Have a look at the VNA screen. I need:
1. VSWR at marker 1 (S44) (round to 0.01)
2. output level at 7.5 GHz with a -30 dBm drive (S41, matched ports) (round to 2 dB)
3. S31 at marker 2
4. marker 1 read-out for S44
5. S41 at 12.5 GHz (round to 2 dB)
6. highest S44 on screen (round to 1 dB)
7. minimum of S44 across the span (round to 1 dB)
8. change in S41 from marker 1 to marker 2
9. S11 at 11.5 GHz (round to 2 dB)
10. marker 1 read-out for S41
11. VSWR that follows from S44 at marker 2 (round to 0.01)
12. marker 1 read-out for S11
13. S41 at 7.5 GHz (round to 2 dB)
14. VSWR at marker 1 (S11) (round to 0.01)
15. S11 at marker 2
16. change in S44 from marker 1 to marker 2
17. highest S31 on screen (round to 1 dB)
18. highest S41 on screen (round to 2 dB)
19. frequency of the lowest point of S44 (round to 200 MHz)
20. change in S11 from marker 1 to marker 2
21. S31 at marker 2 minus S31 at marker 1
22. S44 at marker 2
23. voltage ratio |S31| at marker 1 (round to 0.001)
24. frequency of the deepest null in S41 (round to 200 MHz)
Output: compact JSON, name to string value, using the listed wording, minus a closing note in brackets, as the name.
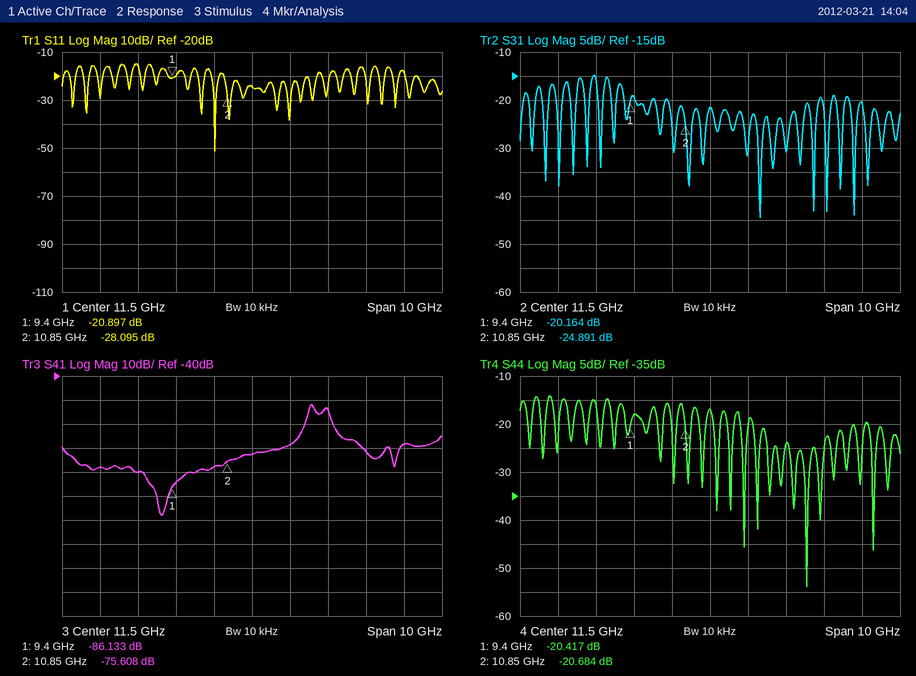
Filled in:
{"VSWR at marker 1 (S44)": "1.21", "output level at 7.5 GHz with a -30 dBm drive (S41, matched ports)": "-108 dBm", "S31 at marker 2": "-24.891 dB", "marker 1 read-out for S44": "-20.417 dB", "S41 at 12.5 GHz": "-68 dB", "highest S44 on screen": "-14 dB", "minimum of S44 across the span": "-54 dB", "change in S41 from marker 1 to marker 2": "10.525 dB", "S11 at 11.5 GHz": "-24 dB", "marker 1 read-out for S41": "-86.133 dB", "VSWR that follows from S44 at marker 2": "1.20", "marker 1 read-out for S11": "-20.897 dB", "S41 at 7.5 GHz": "-78 dB", "VSWR at marker 1 (S11)": "1.20", "S11 at marker 2": "-28.095 dB", "change in S44 from marker 1 to marker 2": "-0.267 dB", "highest S31 on screen": "-15 dB", "highest S41 on screen": "-52 dB", "frequency of the lowest point of S44": "14.0 GHz", "change in S11 from marker 1 to marker 2": "-7.198 dB", "S31 at marker 2 minus S31 at marker 1": "-4.727 dB", "S44 at marker 2": "-20.684 dB", "voltage ratio |S31| at marker 1": "0.098", "frequency of the deepest null in S41": "9.2 GHz"}
